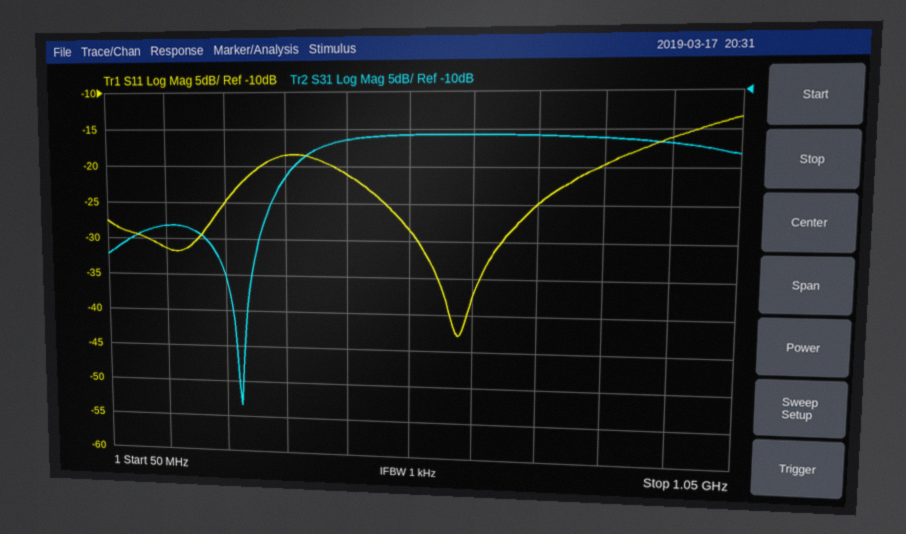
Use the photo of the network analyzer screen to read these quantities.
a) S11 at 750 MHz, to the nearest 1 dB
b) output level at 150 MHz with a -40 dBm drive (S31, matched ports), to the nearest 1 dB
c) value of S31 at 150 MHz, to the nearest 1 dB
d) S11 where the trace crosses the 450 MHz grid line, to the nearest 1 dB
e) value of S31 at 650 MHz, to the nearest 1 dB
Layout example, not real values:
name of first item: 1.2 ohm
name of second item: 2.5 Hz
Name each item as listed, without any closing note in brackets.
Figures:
S11 at 750 MHz, to the nearest 1 dB: -25 dB
output level at 150 MHz with a -40 dBm drive (S31, matched ports), to the nearest 1 dB: -68 dBm
value of S31 at 150 MHz, to the nearest 1 dB: -28 dB
S11 where the trace crosses the 450 MHz grid line, to the nearest 1 dB: -21 dB
value of S31 at 650 MHz, to the nearest 1 dB: -16 dB
